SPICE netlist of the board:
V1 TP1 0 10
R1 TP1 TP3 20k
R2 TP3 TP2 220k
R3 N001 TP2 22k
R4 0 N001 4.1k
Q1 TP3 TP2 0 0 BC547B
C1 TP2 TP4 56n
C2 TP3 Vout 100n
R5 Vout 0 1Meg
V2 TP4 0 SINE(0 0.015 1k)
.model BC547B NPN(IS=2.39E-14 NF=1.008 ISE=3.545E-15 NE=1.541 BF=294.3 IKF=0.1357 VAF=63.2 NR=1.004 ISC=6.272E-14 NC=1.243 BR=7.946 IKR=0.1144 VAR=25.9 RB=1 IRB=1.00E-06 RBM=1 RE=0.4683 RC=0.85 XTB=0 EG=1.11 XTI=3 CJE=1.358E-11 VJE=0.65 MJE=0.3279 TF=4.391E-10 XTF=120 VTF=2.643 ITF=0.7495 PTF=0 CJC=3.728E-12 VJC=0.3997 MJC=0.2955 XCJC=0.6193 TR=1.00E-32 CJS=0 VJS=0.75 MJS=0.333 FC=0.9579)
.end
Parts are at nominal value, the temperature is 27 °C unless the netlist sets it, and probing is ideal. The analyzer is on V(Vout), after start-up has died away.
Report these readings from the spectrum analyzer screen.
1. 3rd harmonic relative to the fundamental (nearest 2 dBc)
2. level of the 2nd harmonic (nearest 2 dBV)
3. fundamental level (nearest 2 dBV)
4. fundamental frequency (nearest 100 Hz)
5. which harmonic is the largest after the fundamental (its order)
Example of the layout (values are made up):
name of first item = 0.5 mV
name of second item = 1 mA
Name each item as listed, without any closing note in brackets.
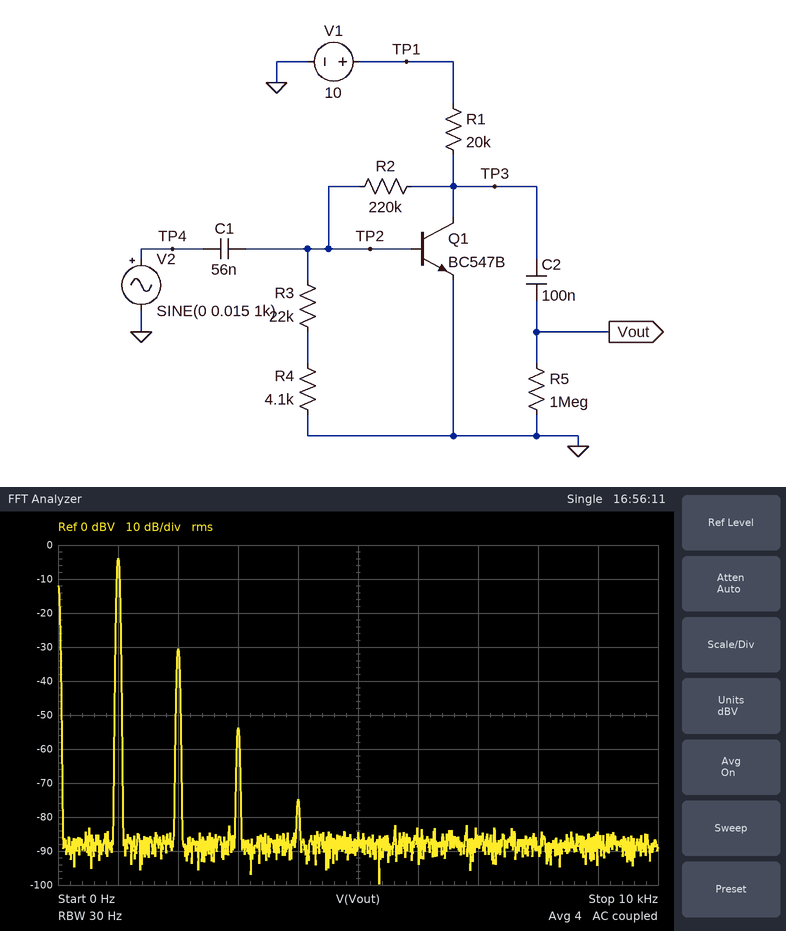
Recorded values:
3rd harmonic relative to the fundamental = -50 dBc
level of the 2nd harmonic = -30 dBV
fundamental level = -4 dBV
fundamental frequency = 1.0 kHz
which harmonic is the largest after the fundamental = 2
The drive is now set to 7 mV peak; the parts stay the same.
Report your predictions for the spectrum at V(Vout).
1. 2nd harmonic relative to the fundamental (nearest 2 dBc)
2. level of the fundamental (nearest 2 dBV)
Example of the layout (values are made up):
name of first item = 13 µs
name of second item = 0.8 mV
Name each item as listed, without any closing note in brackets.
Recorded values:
2nd harmonic relative to the fundamental = -34 dBc
level of the fundamental = -10 dBV
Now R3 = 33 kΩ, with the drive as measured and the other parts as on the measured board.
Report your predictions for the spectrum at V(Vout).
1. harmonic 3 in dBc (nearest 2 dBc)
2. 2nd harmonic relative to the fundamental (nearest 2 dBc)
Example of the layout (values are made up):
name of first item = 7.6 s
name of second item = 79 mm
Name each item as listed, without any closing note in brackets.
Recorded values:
harmonic 3 in dBc = -54 dBc
2nd harmonic relative to the fundamental = -30 dBc
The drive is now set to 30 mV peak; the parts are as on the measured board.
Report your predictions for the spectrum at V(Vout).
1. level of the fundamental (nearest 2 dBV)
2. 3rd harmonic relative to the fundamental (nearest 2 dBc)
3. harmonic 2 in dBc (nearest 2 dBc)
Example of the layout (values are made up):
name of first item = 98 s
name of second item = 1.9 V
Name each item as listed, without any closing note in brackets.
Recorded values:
level of the fundamental = 2 dBV
3rd harmonic relative to the fundamental = -38 dBc
harmonic 2 in dBc = -20 dBc
